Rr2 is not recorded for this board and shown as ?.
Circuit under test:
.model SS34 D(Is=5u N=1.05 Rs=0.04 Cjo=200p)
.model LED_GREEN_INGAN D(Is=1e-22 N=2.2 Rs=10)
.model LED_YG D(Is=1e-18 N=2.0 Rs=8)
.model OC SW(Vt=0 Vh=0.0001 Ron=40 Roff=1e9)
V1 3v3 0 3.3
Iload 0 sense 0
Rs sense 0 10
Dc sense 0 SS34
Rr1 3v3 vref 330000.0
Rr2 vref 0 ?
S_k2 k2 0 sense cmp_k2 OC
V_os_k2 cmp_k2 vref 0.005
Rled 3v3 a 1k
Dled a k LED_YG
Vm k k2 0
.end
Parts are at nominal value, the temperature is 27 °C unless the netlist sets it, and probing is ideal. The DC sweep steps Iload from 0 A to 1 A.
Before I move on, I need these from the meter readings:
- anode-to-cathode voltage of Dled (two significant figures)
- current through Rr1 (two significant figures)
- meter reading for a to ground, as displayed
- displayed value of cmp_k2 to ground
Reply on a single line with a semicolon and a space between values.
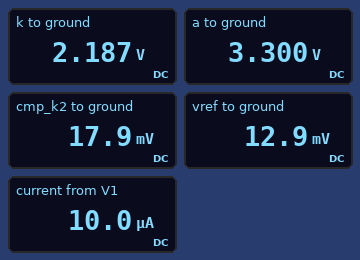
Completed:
1.1 V; 10 µA; 3.300 V; 17.9 mV
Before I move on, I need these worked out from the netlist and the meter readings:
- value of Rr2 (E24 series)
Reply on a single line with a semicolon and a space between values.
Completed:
1.3 kΩ
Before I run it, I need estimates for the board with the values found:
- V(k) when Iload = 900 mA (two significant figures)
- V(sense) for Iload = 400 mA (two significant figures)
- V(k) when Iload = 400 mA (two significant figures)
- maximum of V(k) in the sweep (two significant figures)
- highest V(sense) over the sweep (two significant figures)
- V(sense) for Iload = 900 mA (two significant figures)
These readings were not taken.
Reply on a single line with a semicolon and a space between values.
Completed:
57 mV; 320 mV; 57 mV; 2.2 V; 370 mV; 360 mV
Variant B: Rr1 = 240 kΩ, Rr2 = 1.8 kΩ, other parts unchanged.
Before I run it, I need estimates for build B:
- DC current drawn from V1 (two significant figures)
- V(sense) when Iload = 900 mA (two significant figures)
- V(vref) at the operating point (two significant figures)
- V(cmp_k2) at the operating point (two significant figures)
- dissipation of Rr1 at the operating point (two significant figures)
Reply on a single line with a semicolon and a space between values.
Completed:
14 µA; 360 mV; 25 mV; 30 mV; 45 µW
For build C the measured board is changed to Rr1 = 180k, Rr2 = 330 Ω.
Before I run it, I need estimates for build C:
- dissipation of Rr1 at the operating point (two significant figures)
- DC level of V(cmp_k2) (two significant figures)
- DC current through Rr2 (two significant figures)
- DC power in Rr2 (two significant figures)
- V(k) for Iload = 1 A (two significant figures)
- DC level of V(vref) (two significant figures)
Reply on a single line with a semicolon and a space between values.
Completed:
60 µW; 11 mV; 18 µA; 110 nW; 57 mV; 6.0 mV
